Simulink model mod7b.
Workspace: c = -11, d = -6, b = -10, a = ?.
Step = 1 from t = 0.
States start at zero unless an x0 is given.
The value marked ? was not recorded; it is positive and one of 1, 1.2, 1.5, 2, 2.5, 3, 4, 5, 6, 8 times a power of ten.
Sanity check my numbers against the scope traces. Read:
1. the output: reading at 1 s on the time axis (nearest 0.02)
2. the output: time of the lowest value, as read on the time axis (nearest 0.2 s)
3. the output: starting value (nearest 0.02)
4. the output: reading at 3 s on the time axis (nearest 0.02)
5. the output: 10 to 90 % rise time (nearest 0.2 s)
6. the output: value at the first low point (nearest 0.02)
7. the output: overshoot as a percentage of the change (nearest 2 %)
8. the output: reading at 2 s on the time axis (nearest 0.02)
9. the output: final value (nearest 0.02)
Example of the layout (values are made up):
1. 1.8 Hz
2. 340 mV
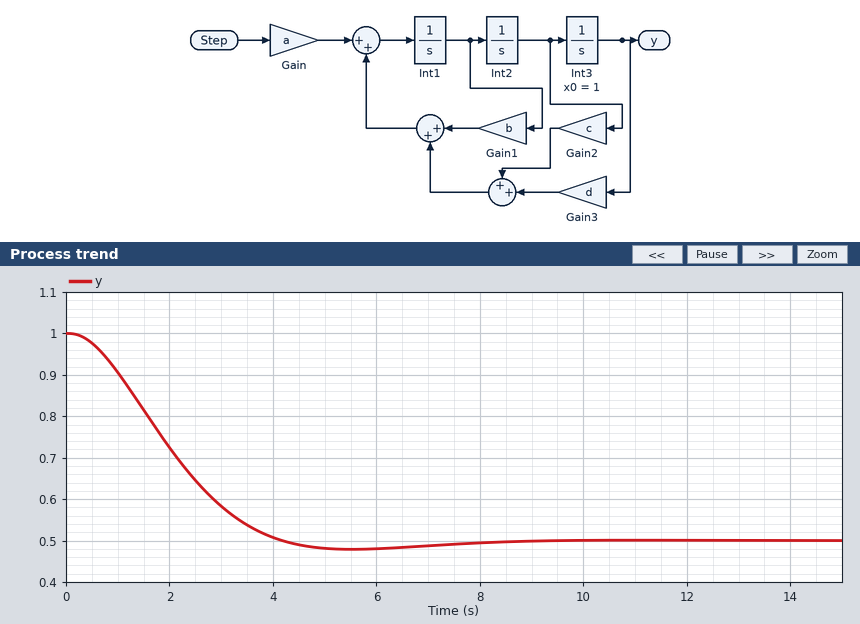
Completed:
1. 0.90
2. 5.6 s
3. 1.00
4. 0.58
5. 2.6 s
6. 0.48
7. 4 %
8. 0.72
9. 0.50
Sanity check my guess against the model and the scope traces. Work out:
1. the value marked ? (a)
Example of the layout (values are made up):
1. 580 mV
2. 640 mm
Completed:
1. 3
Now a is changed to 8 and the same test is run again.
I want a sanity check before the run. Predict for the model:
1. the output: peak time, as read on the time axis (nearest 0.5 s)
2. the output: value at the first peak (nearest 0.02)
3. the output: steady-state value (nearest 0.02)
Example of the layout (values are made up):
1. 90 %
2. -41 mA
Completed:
1. 5.5 s
2. 1.34
3. 1.34
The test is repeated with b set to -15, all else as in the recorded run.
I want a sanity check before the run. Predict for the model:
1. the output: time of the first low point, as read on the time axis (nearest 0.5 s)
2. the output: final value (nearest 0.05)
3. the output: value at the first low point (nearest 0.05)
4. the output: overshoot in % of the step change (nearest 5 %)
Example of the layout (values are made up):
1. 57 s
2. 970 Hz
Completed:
1. 6.0 s
2. 0.50
3. 0.45
4. 10 %
